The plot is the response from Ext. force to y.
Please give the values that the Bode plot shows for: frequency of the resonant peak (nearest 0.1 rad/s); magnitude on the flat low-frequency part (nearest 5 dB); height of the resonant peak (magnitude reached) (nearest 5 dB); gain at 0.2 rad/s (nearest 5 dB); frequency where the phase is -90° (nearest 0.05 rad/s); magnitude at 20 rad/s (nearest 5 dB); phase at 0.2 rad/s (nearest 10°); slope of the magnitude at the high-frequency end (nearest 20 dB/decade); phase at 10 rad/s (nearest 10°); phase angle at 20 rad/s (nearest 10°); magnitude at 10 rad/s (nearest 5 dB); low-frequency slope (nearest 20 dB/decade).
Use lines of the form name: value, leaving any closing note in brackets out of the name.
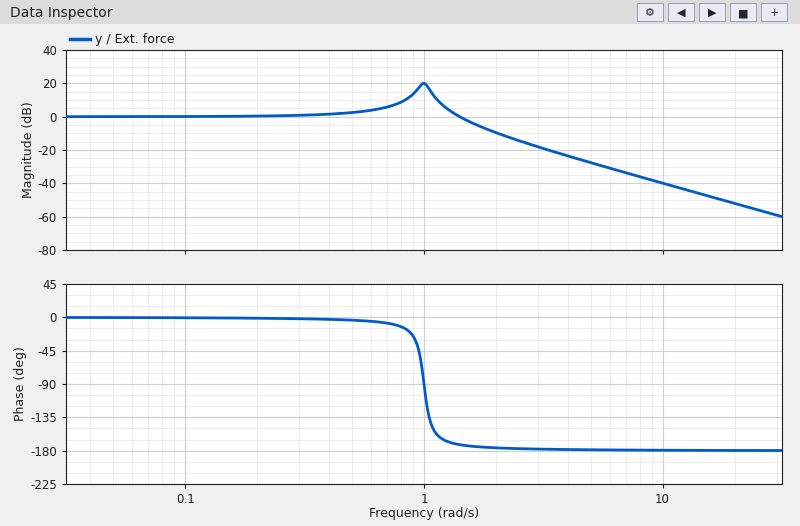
frequency of the resonant peak: 1.0 rad/s
magnitude on the flat low-frequency part: 0 dB
height of the resonant peak (magnitude reached): 20 dB
gain at 0.2 rad/s: 0 dB
frequency where the phase is -90°: 1.00 rad/s
magnitude at 20 rad/s: -50 dB
phase at 0.2 rad/s: 0°
slope of the magnitude at the high-frequency end: -40 dB/decade
phase at 10 rad/s: -180°
phase angle at 20 rad/s: -180°
magnitude at 10 rad/s: -40 dB
low-frequency slope: 0 dB/decade
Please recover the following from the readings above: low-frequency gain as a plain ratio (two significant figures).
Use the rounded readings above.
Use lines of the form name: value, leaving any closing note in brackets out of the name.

low-frequency gain as a plain ratio: 1.0
